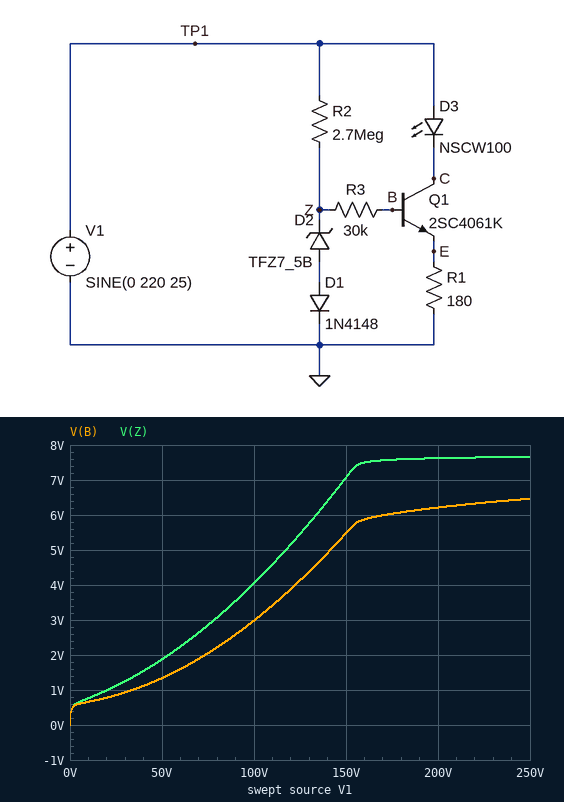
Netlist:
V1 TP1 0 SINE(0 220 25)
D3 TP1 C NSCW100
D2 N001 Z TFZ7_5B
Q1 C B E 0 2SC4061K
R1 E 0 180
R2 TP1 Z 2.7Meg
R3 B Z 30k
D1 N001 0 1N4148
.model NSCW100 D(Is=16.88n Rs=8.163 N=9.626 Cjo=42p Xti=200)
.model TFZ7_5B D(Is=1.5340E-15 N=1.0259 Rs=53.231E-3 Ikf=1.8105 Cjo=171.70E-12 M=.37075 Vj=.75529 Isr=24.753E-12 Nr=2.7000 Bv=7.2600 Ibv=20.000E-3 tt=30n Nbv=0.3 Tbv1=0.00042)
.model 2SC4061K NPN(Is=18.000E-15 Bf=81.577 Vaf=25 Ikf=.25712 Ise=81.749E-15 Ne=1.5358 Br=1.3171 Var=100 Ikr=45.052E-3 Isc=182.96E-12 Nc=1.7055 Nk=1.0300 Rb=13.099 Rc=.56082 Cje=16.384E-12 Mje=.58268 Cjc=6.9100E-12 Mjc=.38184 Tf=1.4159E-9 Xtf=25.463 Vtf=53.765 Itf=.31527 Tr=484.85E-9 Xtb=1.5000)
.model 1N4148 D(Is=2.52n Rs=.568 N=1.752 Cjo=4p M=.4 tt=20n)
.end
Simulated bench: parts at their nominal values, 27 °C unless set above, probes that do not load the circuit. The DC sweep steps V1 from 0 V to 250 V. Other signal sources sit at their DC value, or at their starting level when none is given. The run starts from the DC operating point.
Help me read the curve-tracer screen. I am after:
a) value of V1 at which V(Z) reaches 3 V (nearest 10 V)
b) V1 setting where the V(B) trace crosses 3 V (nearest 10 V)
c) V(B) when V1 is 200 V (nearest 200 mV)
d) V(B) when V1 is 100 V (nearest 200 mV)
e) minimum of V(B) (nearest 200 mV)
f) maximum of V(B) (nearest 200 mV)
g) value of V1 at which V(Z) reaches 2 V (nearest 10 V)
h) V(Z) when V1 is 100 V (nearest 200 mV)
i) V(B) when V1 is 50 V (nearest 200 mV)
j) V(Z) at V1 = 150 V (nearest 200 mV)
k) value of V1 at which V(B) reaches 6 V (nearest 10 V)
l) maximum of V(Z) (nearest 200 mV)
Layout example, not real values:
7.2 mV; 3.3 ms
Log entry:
80 V; 100 V; 6.2 V; 3.0 V; 0 V; 6.4 V; 50 V; 4.0 V; 1.4 V; 7.0 V; 170 V; 7.6 V
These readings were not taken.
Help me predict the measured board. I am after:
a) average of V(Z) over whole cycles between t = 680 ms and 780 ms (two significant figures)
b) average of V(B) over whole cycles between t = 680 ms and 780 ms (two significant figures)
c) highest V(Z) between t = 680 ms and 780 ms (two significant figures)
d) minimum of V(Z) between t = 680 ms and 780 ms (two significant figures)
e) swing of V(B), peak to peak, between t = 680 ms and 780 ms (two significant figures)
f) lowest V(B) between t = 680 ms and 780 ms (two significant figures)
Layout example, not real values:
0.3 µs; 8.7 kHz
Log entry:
-67 V; -68 V; 7.6 V; -220 V; 230 V; -220 V
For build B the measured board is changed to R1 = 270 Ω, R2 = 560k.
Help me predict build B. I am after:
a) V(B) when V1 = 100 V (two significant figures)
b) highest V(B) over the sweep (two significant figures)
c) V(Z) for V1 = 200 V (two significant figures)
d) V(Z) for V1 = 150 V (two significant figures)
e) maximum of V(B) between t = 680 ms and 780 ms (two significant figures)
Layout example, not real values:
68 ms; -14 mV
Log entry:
6.0 V; 6.9 V; 7.8 V; 7.7 V; 6.8 V
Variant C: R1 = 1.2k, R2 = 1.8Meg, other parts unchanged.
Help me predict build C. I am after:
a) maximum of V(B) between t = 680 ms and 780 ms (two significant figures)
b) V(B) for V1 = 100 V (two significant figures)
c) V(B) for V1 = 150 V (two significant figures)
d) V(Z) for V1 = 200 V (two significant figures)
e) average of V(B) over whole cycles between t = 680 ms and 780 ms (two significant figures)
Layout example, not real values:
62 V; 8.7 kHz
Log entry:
7.5 V; 7.2 V; 7.3 V; 7.7 V; -67 V
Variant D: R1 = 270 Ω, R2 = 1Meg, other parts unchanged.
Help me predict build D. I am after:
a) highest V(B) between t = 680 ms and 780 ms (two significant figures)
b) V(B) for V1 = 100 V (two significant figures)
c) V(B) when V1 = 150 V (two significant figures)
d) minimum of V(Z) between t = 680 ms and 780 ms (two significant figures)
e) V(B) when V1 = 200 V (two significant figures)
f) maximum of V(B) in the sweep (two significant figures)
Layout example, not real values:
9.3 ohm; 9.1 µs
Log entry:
6.8 V; 6.0 V; 6.4 V; -220 V; 6.7 V; 6.9 V
